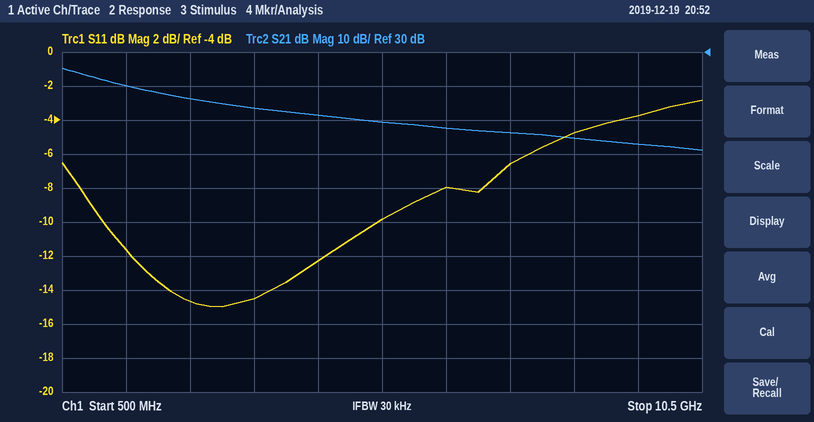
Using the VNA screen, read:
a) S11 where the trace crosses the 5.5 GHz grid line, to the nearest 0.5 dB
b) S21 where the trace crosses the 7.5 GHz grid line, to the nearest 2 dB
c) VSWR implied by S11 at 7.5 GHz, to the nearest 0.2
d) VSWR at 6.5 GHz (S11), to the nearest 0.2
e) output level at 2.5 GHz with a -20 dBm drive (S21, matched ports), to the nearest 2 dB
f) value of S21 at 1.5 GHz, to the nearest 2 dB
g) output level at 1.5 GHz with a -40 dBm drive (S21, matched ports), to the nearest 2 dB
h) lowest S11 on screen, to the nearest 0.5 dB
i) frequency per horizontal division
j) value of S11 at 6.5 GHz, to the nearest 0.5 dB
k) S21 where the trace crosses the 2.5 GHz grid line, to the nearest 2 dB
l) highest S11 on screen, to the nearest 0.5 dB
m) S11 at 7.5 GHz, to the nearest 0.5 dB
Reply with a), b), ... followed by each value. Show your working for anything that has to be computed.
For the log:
a) -10.0 dB
b) 6 dB
c) |Γ| = 10^(-6.5/20) = 0.4732; VSWR = (1 + 0.4732)/(1 − 0.4732) ≈ 2.8
d) |Γ| = 10^(-8/20) = 0.3981; VSWR = (1 + 0.3981)/(1 − 0.3981) ≈ 2.32, so 2.4 to the nearest 0.2
e) -20 dBm + (16 dB) = -4 dBm
f) 20 dB
g) -40 dBm + (20 dB) = -20 dBm
h) -15.0 dB
i) 1 GHz
j) -8.0 dB
k) 16 dB
l) -3.0 dB
m) -6.5 dB
